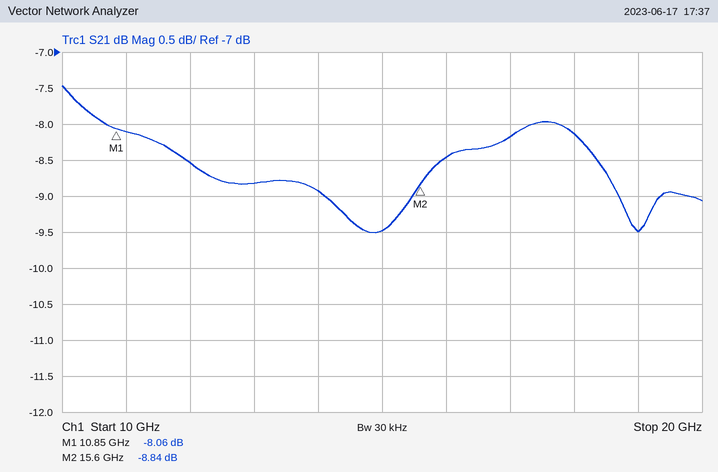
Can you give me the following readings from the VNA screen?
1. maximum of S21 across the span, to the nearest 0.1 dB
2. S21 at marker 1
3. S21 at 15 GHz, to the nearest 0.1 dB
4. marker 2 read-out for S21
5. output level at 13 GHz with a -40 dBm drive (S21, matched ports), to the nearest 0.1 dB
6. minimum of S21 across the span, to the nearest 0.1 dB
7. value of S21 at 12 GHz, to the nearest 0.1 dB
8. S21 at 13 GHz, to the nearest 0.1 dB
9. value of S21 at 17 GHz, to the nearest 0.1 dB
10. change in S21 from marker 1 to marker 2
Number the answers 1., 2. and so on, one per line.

1. -7.5 dB
2. -8.06 dB
3. -9.5 dB
4. -8.84 dB
5. -48.8 dBm
6. -9.5 dB
7. -8.5 dB
8. -8.8 dB
9. -8.2 dB
10. -0.78 dB
